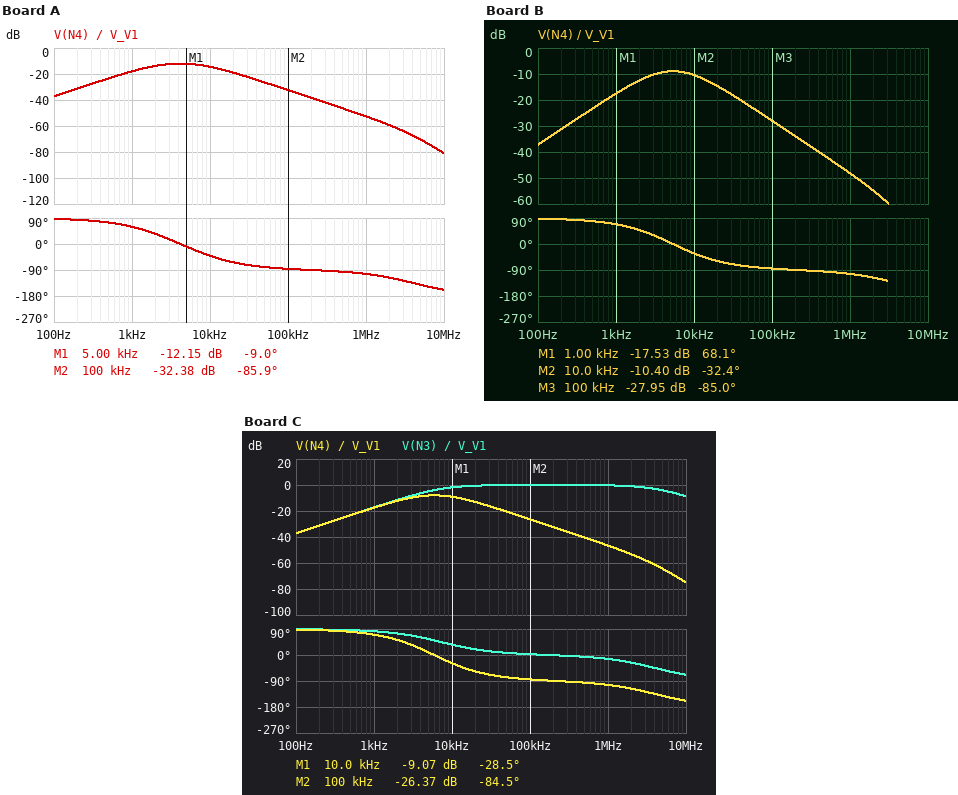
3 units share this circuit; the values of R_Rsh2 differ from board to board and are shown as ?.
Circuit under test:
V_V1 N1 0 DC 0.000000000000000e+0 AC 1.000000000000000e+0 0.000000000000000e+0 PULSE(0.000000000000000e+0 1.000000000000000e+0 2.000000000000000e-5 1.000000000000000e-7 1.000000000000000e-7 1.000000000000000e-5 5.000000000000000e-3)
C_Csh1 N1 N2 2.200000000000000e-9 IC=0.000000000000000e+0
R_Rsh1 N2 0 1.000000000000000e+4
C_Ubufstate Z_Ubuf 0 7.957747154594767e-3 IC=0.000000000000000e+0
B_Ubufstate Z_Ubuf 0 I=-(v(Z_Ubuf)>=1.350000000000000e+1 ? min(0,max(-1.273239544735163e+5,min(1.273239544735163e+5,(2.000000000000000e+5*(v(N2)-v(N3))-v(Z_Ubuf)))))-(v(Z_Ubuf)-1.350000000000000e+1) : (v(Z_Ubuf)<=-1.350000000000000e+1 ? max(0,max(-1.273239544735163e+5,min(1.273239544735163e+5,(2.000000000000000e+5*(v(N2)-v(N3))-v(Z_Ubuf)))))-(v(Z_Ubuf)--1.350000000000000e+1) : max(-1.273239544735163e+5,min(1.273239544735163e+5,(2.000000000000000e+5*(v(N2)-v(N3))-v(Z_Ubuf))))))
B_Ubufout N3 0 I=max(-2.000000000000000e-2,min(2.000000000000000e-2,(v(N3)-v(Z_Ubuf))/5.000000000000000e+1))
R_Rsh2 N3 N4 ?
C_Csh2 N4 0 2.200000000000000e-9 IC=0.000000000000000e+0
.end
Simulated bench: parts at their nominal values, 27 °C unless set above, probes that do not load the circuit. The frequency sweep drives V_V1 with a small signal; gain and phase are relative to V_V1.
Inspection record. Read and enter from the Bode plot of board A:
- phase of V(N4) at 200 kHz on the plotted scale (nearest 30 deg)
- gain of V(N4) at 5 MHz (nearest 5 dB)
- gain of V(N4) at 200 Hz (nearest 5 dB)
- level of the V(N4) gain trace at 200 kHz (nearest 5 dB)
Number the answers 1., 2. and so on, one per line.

1. -90 deg
2. -70 dB
3. -30 dB
4. -40 dB
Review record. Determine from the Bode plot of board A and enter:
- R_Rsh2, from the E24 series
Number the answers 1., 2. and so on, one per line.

1. 30 kΩ
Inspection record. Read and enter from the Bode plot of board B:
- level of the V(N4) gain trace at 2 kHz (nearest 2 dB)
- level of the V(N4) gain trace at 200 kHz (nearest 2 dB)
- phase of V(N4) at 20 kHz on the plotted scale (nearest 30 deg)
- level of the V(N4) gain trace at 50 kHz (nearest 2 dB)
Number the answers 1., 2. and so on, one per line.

1. -12 dB
2. -34 dB
3. -60 deg
4. -22 dB
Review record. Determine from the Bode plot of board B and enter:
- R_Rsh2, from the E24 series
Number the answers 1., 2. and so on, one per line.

1. 18 kΩ
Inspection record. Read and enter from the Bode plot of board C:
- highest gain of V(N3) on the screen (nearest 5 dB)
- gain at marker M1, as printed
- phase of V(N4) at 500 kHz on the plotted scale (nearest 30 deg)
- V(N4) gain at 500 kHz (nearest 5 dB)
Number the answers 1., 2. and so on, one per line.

1. 0 dB
2. -9.07 dB
3. -90 deg
4. -40 dB
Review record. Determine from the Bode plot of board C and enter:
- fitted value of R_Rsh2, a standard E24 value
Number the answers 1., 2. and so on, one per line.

1. 15 kΩ
